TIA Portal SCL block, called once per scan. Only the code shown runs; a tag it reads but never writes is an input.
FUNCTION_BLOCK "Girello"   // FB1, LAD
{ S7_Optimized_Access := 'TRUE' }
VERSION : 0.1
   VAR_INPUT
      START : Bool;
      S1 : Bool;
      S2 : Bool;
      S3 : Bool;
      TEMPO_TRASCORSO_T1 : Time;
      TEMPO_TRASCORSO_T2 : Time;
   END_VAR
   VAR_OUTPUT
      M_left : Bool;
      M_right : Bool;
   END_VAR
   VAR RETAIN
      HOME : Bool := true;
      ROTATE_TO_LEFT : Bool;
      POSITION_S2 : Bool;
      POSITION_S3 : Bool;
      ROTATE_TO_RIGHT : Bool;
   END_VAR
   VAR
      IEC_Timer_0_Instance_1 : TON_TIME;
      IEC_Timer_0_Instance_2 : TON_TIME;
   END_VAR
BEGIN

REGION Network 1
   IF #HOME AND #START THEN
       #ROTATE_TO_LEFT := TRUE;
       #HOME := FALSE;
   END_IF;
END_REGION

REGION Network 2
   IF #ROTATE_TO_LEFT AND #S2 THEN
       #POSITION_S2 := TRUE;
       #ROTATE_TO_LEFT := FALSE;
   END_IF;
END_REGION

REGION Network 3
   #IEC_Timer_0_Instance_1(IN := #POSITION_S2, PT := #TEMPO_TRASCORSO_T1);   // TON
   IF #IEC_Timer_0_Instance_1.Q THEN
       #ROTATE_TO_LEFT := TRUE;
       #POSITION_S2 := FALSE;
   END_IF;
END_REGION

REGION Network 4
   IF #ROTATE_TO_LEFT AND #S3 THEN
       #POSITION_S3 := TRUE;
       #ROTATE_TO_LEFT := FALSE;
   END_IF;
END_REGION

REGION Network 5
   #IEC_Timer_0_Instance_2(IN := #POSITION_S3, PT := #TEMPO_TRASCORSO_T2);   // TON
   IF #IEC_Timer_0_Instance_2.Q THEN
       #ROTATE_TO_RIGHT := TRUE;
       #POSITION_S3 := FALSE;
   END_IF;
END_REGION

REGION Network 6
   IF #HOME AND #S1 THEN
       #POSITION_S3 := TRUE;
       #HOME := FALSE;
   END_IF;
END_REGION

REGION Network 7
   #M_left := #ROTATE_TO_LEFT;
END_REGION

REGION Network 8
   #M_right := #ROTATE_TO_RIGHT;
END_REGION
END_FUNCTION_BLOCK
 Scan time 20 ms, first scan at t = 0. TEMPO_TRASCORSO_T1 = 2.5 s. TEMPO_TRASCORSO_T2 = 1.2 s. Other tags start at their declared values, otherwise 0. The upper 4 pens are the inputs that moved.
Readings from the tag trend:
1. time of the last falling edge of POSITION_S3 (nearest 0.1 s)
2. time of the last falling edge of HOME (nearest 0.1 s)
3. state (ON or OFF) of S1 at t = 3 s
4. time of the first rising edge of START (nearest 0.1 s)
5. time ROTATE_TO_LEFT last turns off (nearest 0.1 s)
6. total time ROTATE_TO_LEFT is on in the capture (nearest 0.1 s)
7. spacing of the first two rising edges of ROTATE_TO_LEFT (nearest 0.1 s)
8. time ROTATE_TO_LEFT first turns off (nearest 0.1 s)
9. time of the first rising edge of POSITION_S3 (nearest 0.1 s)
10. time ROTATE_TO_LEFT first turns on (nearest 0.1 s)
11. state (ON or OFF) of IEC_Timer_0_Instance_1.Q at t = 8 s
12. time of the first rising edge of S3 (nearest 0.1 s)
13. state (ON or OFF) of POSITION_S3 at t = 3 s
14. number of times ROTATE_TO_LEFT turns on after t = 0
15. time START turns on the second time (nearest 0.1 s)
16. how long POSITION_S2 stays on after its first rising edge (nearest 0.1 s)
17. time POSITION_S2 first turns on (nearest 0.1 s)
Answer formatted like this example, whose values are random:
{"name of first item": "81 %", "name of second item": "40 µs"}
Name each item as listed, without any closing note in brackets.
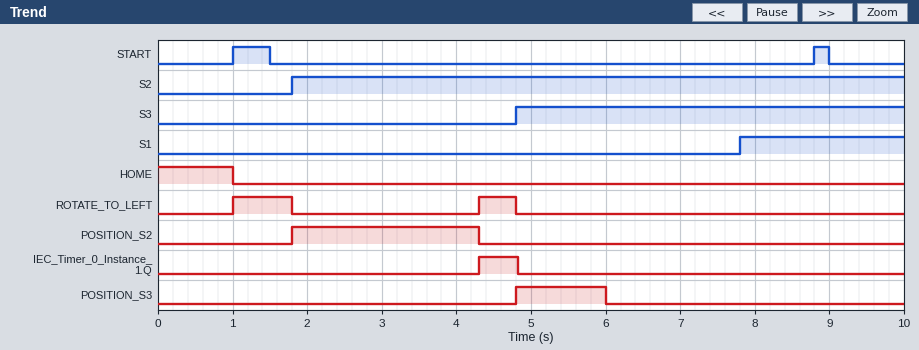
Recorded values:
{"time of the last falling edge of POSITION_S3": "6.0 s", "time of the last falling edge of HOME": "1.0 s", "state (ON or OFF) of S1 at t = 3 s": "OFF", "time of the first rising edge of START": "1.0 s", "time ROTATE_TO_LEFT last turns off": "4.8 s", "total time ROTATE_TO_LEFT is on in the capture": "1.3 s", "spacing of the first two rising edges of ROTATE_TO_LEFT": "3.3 s", "time ROTATE_TO_LEFT first turns off": "1.8 s", "time of the first rising edge of POSITION_S3": "4.8 s", "time ROTATE_TO_LEFT first turns on": "1.0 s", "state (ON or OFF) of IEC_Timer_0_Instance_1.Q at t = 8 s": "OFF", "time of the first rising edge of S3": "4.8 s", "state (ON or OFF) of POSITION_S3 at t = 3 s": "OFF", "number of times ROTATE_TO_LEFT turns on after t = 0": "2", "time START turns on the second time": "8.8 s", "how long POSITION_S2 stays on after its first rising edge": "2.5 s", "time POSITION_S2 first turns on": "1.8 s"}
